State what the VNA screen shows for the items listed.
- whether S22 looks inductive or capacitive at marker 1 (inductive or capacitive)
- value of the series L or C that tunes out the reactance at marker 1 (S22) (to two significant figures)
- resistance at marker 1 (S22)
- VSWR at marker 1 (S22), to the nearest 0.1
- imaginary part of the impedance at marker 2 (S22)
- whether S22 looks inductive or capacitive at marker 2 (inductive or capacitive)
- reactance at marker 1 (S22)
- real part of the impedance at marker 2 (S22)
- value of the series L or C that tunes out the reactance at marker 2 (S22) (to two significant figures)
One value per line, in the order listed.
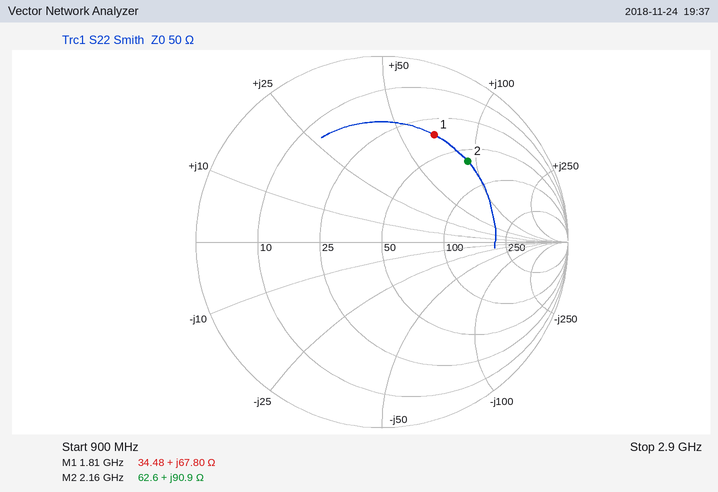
inductive
1.3 pF
34.48 Ω
4.6
+90.9 Ω
inductive
+67.80 Ω
62.6 Ω
810 fF
